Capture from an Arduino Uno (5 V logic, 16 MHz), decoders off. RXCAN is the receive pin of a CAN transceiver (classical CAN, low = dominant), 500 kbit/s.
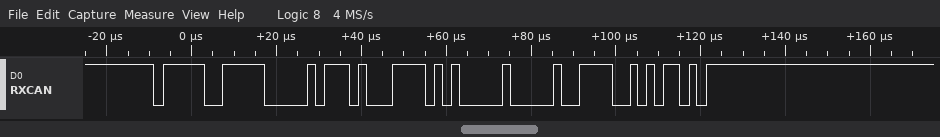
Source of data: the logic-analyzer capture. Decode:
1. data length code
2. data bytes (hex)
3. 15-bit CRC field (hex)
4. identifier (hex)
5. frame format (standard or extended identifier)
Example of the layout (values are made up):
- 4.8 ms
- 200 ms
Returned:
- 3
- A3 D4 00
- 0x1E56
- 0x7DF
- standard
